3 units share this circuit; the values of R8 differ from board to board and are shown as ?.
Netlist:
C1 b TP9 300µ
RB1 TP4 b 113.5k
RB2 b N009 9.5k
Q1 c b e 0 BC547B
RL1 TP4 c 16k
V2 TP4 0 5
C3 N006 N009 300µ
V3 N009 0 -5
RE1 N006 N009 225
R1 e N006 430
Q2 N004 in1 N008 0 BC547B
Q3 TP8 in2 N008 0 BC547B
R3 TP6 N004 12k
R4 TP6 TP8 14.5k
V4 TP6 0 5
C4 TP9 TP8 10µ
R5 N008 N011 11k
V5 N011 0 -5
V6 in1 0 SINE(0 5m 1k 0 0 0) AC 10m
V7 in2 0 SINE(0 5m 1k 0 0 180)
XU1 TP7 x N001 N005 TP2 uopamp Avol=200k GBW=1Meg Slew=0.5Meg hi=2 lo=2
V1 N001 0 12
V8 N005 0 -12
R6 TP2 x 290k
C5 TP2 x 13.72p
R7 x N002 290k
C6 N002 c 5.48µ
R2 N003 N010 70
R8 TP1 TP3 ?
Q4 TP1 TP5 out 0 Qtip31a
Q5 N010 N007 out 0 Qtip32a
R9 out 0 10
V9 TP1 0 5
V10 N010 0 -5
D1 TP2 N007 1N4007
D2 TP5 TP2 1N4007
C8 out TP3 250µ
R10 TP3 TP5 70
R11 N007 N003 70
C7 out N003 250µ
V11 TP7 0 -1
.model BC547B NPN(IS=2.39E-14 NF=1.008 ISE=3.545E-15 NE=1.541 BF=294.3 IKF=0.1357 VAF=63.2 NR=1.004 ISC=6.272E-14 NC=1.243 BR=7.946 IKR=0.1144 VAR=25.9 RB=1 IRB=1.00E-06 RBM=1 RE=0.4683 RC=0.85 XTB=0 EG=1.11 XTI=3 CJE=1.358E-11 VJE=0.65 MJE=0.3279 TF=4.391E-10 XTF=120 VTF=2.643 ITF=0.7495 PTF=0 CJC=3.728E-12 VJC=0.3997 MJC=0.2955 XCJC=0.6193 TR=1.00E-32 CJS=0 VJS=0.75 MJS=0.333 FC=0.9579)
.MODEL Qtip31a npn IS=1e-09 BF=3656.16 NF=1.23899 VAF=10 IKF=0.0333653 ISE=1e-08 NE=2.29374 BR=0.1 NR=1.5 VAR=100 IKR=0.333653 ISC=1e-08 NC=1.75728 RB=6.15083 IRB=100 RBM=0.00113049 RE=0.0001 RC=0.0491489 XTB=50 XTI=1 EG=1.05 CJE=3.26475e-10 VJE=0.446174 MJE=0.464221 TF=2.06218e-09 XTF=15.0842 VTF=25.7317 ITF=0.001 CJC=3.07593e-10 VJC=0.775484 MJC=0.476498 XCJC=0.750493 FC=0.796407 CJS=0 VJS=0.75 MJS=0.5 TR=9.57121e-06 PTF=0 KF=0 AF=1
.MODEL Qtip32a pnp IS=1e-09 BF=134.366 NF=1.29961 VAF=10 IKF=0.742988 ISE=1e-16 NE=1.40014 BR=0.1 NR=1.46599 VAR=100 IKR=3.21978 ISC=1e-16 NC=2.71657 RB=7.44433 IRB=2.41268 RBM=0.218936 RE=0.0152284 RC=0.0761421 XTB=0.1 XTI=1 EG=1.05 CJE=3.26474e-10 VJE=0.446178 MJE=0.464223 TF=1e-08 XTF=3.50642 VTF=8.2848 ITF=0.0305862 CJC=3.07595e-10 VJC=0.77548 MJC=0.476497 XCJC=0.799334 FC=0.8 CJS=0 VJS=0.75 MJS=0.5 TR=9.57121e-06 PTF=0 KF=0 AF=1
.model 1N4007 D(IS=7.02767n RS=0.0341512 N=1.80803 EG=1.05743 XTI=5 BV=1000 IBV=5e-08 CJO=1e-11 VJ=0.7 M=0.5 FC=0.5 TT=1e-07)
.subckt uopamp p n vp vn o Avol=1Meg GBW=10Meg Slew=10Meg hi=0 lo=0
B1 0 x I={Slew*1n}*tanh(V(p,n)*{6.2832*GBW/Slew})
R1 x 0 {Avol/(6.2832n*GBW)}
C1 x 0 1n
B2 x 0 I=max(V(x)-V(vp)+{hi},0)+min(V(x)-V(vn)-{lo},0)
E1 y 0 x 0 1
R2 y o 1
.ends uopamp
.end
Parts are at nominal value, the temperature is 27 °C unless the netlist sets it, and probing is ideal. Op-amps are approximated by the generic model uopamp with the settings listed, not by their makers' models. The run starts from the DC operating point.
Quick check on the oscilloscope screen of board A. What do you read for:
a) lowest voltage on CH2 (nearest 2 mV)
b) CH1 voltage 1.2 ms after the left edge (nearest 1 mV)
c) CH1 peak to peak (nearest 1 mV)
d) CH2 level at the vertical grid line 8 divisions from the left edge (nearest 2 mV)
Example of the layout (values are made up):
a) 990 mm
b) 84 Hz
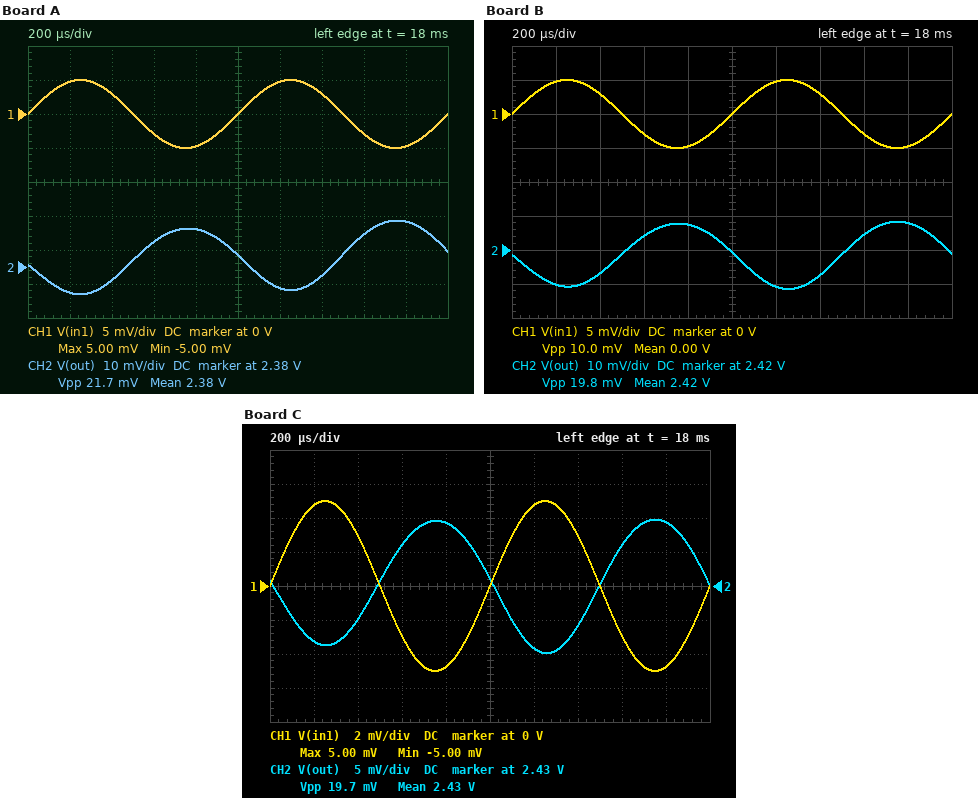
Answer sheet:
a) 2.372 V
b) 5 mV
c) 10 mV
d) 2.390 V
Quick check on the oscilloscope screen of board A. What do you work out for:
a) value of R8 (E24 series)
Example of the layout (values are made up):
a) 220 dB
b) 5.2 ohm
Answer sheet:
a) 200 Ω
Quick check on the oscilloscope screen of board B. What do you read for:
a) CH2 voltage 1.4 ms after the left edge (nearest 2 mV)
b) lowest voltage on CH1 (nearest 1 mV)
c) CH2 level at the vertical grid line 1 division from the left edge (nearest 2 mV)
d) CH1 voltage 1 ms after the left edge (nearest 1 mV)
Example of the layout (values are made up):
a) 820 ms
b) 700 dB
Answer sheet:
a) 2.412 V
b) -5 mV
c) 2.410 V
d) 0 V
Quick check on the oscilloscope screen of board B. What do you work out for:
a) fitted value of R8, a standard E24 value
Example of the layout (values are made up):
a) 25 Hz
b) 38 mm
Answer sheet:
a) 75 Ω
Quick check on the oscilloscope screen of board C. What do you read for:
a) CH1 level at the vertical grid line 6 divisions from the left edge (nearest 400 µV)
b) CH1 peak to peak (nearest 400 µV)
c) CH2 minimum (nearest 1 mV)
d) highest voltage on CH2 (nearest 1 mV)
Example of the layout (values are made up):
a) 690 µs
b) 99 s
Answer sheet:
a) 4.8 mV
b) 10.0 mV
c) 2.420 V
d) 2.440 V
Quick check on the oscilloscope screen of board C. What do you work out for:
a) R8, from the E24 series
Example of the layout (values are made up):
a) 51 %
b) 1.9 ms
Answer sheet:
a) 39 Ω
